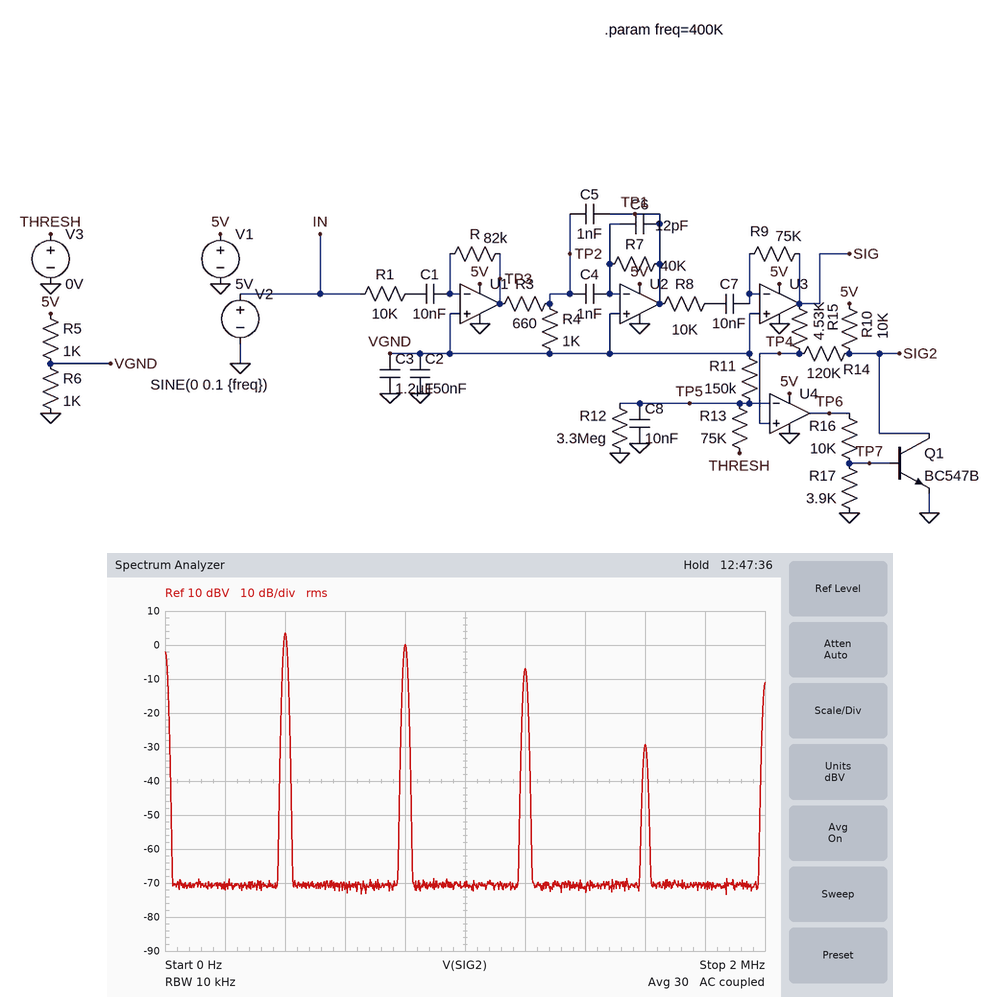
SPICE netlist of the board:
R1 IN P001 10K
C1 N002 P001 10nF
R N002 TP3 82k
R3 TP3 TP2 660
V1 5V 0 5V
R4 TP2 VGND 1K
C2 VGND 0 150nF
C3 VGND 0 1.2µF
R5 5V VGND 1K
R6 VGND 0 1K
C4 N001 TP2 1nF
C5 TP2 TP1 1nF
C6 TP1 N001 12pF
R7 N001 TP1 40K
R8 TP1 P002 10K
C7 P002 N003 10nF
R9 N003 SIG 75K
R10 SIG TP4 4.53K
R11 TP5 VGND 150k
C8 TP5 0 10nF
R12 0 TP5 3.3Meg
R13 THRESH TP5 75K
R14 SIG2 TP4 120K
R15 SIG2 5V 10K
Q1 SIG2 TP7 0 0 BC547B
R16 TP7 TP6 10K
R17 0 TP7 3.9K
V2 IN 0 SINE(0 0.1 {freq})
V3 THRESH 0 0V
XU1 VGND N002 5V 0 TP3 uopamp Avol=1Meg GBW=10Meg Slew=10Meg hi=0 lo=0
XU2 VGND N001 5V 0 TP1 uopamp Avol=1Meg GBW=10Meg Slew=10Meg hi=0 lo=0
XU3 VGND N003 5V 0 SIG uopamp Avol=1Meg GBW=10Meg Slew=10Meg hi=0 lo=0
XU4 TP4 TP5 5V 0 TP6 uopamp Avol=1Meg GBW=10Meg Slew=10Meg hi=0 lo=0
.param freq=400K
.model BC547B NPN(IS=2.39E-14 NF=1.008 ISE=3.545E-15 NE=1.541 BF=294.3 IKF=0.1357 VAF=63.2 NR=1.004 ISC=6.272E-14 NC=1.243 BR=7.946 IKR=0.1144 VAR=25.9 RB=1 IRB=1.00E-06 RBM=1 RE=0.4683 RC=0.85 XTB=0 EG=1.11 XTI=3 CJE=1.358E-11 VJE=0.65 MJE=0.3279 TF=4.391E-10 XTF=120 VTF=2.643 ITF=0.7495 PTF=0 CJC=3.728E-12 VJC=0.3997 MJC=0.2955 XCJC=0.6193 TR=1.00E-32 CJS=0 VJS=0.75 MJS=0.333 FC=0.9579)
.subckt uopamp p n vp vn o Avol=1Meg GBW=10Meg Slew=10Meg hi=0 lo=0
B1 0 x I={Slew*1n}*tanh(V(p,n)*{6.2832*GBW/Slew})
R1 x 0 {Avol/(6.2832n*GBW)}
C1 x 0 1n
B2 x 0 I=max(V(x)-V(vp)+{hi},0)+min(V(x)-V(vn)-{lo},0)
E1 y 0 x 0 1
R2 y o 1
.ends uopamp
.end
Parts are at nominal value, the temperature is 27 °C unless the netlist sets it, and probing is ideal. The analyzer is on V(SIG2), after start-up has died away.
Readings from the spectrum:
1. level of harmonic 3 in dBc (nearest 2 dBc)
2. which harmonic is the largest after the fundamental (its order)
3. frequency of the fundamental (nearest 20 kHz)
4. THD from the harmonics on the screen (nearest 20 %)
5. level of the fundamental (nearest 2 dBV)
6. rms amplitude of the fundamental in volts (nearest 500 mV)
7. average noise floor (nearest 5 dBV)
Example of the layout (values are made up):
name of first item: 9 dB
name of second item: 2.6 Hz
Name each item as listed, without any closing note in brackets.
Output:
level of harmonic 3 in dBc: -10 dBc
which harmonic is the largest after the fundamental: 2
frequency of the fundamental: 400 kHz
THD from the harmonics on the screen: 80 %
level of the fundamental: 4 dBV
rms amplitude of the fundamental in volts: 1.5 V
average noise floor: -70 dBV
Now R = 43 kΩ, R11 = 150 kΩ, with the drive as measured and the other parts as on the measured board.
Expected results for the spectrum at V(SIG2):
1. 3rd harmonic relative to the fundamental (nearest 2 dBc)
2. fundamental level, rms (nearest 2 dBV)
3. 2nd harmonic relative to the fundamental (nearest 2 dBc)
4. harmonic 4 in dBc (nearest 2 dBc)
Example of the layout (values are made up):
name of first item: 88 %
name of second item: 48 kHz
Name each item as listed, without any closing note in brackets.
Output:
3rd harmonic relative to the fundamental: 10 dBc
fundamental level, rms: -90 dBV
2nd harmonic relative to the fundamental: 12 dBc
harmonic 4 in dBc: 10 dBc
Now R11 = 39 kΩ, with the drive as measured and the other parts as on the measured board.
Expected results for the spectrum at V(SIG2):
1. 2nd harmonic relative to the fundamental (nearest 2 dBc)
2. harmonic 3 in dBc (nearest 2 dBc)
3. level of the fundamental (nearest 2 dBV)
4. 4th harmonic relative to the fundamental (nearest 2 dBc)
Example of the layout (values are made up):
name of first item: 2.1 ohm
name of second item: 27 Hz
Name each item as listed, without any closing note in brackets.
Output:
2nd harmonic relative to the fundamental: -8 dBc
harmonic 3 in dBc: -22 dBc
level of the fundamental: 6 dBV
4th harmonic relative to the fundamental: -12 dBc
